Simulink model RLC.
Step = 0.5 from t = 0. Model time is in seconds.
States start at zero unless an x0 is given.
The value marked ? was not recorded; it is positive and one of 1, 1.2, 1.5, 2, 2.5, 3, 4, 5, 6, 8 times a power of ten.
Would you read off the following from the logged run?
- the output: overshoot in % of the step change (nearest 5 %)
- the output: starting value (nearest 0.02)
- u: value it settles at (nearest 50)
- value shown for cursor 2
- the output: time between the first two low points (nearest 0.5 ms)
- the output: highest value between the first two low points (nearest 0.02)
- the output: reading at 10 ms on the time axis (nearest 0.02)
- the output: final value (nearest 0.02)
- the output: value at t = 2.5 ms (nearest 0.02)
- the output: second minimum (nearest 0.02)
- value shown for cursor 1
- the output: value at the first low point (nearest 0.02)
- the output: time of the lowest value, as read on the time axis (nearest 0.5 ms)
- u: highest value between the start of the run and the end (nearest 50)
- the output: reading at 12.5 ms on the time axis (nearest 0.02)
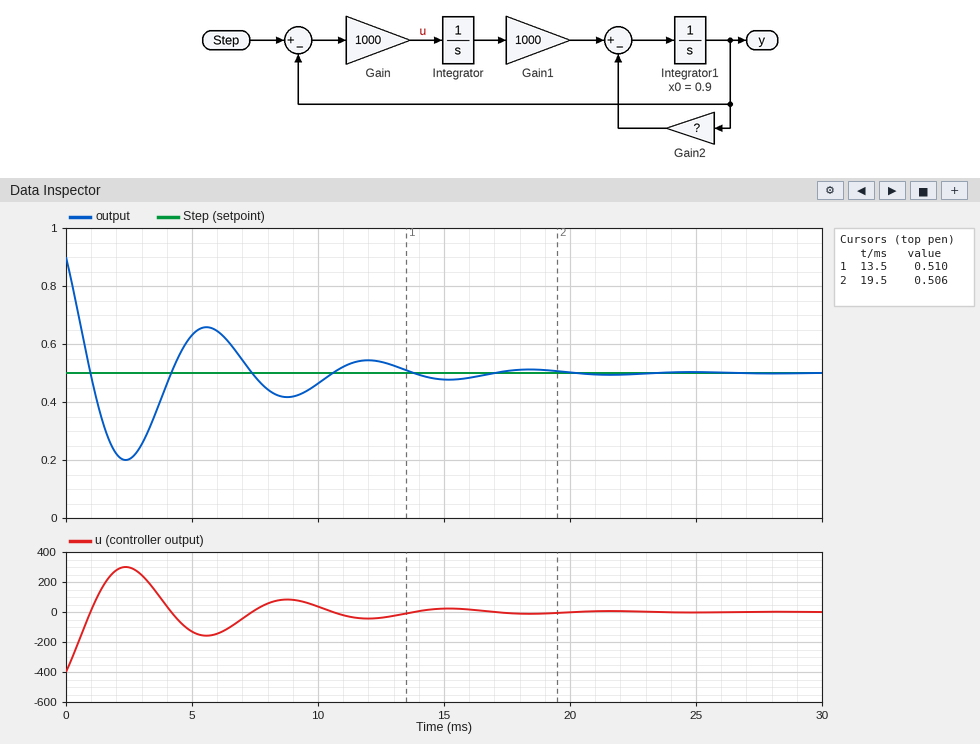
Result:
75 %
0.90
0
0.506
6.5 ms
0.66
0.46
0.50
0.20
0.42
0.510
0.20
2.5 ms
300
0.54
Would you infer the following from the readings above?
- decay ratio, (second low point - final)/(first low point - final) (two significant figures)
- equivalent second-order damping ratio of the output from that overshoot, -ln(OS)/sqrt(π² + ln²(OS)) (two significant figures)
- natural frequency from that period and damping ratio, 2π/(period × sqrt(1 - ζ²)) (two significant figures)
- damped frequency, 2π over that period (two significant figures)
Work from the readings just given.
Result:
0.27
0.091
0.97 rad/ms
0.97 rad/ms
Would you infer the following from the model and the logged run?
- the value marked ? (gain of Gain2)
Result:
400
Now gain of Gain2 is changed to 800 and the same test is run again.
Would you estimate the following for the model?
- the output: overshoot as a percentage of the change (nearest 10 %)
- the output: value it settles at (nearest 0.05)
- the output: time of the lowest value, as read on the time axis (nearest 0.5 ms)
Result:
80 %
0.50
2.0 ms
